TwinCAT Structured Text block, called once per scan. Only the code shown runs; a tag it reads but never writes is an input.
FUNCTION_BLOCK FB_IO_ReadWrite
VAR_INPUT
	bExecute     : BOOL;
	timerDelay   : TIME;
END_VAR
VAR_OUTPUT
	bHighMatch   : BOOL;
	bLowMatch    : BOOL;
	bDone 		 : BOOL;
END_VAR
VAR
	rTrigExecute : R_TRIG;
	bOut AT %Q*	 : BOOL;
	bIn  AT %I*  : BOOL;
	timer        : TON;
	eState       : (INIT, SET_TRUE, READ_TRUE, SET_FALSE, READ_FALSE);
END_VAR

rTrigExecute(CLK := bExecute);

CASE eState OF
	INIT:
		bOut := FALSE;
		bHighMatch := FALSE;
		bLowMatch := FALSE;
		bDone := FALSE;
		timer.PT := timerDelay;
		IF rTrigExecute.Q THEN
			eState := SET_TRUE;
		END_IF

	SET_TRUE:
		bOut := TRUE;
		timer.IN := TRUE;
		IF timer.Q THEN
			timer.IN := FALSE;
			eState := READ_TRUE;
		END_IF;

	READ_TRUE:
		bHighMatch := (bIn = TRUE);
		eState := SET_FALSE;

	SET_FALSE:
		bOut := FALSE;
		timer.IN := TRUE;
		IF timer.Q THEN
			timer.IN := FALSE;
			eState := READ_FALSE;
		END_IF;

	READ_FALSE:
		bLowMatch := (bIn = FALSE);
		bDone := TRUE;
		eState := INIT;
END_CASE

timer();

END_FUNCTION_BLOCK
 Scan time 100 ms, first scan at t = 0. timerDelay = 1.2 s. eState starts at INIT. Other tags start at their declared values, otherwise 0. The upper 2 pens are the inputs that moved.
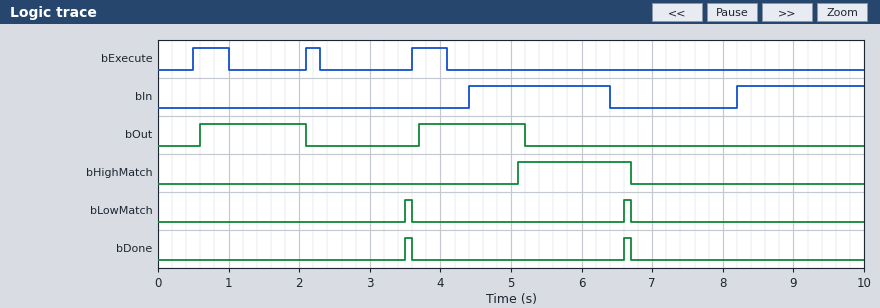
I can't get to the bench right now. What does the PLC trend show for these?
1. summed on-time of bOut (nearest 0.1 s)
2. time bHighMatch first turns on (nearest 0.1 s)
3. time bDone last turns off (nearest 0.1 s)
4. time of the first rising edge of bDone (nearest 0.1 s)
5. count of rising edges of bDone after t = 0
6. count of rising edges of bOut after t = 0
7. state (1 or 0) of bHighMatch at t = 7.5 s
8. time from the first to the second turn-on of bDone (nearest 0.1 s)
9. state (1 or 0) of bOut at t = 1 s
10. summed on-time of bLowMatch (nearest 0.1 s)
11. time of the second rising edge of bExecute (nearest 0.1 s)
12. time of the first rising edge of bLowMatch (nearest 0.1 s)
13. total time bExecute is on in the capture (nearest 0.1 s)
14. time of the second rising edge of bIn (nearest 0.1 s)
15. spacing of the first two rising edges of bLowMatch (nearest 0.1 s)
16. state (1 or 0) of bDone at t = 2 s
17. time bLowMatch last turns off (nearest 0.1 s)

3.0 s
5.1 s
6.7 s
3.5 s
2
2
0
3.1 s
1
0.2 s
2.1 s
3.5 s
1.2 s
8.2 s
3.1 s
0
6.7 s
